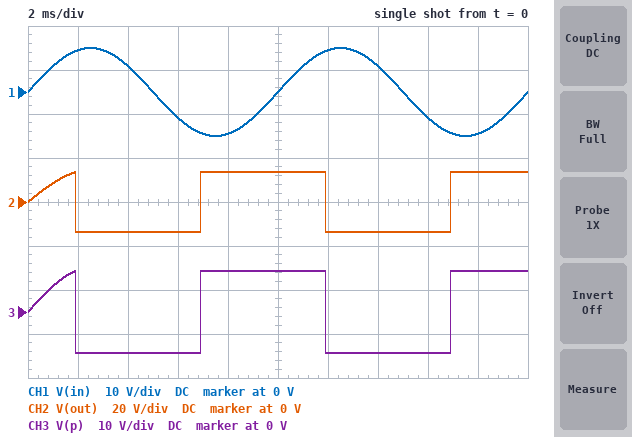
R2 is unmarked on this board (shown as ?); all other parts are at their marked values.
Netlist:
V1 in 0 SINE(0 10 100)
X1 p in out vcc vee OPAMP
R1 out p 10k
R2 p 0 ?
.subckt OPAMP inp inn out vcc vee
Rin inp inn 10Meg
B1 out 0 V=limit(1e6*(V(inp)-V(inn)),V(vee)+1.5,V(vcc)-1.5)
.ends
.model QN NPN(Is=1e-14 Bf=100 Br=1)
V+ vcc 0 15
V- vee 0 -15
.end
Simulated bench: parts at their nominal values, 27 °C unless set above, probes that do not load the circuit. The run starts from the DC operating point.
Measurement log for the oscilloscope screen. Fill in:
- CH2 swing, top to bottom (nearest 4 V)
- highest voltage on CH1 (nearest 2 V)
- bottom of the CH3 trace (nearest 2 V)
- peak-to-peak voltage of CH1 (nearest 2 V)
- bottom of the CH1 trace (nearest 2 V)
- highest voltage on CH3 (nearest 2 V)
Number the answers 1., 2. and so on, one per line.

1. 28 V
2. 10 V
3. -10 V
4. 20 V
5. -10 V
6. 10 V
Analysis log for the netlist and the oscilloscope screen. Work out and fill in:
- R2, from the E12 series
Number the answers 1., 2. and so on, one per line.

1. 22 kΩ
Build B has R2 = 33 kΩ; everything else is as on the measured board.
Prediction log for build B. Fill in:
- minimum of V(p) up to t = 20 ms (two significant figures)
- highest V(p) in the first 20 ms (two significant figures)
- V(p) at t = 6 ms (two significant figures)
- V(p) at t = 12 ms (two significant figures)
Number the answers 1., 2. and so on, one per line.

1. -10 V
2. 10 V
3. -5.9 V
4. 9.5 V
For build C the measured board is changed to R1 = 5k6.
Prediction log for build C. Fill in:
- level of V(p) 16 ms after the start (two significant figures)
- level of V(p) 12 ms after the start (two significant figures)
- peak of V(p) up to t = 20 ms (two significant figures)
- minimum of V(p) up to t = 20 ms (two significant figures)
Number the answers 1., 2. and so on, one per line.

1. -5.9 V
2. 9.5 V
3. 10 V
4. -10 V
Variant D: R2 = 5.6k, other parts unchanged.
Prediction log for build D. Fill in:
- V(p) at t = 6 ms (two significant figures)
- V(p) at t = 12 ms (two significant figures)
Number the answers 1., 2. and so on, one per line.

1. 4.8 V
2. -4.8 V
